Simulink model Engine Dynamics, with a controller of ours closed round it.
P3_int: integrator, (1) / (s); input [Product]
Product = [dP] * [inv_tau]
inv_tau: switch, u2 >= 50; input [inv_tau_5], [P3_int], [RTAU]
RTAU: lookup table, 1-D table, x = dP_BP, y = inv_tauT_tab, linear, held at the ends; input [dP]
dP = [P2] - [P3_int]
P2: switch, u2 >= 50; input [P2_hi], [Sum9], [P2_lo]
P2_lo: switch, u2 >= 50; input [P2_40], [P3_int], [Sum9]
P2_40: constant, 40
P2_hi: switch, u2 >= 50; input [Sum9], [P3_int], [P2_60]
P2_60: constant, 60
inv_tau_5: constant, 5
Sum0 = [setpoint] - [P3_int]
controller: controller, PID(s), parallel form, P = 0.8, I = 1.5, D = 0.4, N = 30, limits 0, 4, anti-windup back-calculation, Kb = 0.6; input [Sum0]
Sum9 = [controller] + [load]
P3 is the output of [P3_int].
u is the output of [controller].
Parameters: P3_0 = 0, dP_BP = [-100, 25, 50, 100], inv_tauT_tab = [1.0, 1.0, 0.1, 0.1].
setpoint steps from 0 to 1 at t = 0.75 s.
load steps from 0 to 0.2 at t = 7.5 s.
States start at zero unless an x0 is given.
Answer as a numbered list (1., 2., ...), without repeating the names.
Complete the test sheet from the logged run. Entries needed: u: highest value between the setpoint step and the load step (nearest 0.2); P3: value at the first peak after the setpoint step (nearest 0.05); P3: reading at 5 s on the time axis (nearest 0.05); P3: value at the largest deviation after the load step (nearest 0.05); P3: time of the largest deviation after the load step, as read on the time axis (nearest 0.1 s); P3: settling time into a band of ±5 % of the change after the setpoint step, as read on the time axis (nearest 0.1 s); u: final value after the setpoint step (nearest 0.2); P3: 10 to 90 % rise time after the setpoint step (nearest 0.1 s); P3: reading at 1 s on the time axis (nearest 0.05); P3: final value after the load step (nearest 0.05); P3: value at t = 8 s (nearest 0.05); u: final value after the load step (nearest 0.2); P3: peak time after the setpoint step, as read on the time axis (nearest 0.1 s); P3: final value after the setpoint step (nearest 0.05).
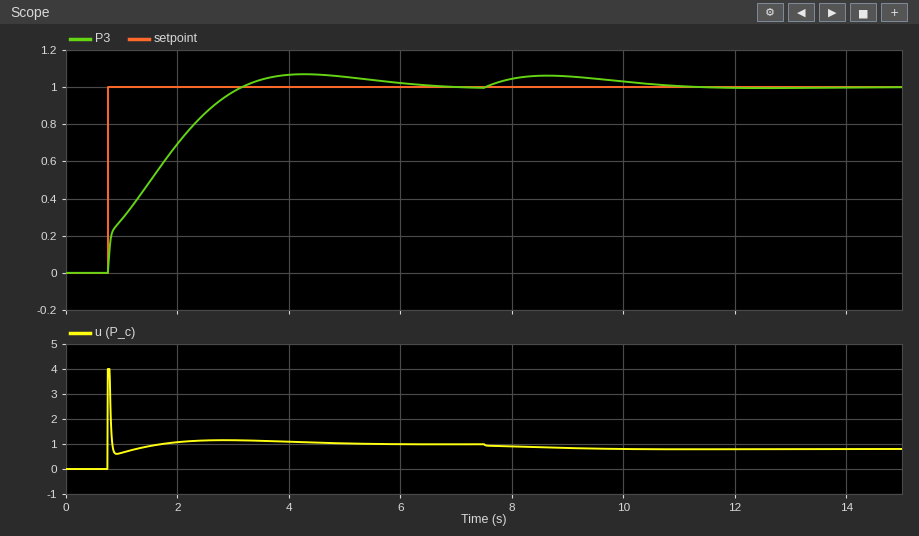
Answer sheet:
1. 4.0
2. 1.05
3. 1.05
4. 1.05
5. 8.6 s
6. 5.2 s
7. 1.0
8. 1.9 s
9. 0.30
10. 1.00
11. 1.05
12. 0.8
13. 4.3 s
14. 1.00
